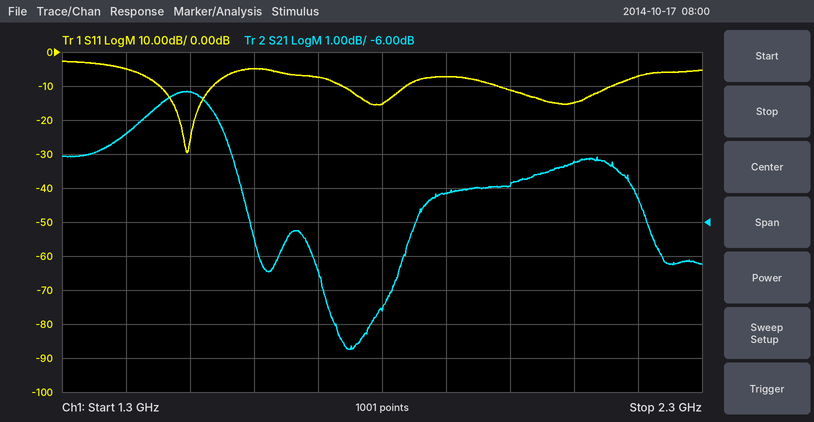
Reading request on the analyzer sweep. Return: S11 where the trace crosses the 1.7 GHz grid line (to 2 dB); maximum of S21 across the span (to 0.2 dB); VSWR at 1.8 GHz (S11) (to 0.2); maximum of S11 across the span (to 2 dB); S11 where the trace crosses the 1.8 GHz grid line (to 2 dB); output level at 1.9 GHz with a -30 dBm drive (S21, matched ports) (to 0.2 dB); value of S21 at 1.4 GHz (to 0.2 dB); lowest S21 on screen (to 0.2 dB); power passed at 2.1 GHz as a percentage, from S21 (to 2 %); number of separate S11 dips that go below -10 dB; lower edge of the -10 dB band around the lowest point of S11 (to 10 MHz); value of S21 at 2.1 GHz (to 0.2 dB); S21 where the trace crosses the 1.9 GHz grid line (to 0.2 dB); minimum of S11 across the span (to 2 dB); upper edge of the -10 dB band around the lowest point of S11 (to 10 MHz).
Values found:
-8 dB
-2.2 dB
1.4
-2 dB
-16 dB
-35.2 dBm
-3.4 dB
-9.8 dB
38 %
3
1.45 GHz
-4.2 dB
-5.2 dB
-30 dB
1.54 GHz
